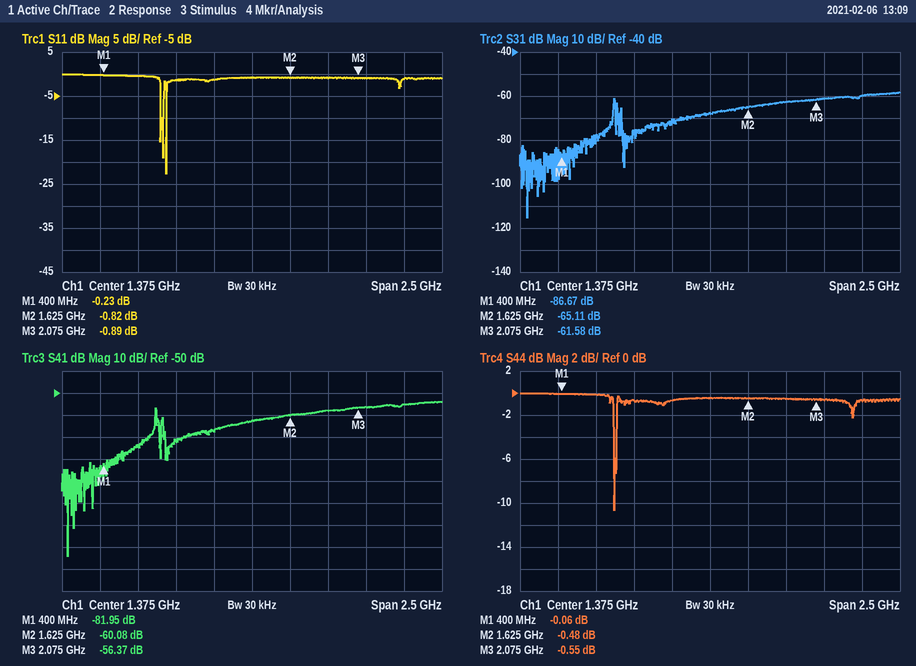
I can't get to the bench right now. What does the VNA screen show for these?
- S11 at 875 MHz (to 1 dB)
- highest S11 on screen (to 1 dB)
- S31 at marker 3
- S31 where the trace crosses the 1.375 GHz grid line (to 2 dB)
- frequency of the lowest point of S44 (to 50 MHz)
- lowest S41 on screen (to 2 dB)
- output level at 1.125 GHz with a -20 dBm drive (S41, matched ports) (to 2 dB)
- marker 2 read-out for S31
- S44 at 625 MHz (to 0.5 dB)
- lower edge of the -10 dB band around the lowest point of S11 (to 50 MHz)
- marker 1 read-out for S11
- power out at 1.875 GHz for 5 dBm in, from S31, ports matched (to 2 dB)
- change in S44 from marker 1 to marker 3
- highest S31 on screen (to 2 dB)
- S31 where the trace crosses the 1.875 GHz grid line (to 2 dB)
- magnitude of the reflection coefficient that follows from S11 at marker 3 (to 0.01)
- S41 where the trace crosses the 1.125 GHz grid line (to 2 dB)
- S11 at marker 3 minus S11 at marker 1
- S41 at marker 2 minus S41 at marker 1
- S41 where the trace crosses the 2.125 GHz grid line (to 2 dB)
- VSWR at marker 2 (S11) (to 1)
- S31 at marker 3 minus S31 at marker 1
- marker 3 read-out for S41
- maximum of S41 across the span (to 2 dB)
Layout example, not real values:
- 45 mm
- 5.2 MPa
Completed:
- -1 dB
- 0 dB
- -61.58 dB
- -68 dB
- 750 MHz
- -124 dB
- -88 dBm
- -65.11 dB
- 0.0 dB
- 800 MHz
- -0.23 dB
- -58 dBm
- -0.49 dB
- -58 dB
- -62 dB
- 0.90
- -68 dB
- -0.66 dB
- 21.87 dB
- -56 dB
- 21
- 25.09 dB
- -56.37 dB
- -54 dB
